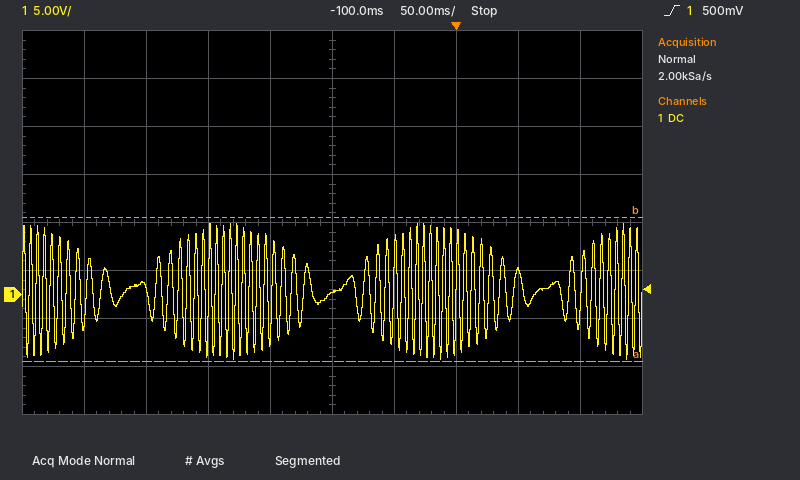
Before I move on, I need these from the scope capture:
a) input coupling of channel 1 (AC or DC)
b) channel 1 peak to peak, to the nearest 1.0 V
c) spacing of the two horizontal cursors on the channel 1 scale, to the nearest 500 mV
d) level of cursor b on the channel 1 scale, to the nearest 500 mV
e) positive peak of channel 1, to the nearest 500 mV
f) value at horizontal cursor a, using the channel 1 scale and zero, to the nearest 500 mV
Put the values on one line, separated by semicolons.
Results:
DC; 14.0 V; 15.0 V; 8.0 V; 7.5 V; -7.0 V
